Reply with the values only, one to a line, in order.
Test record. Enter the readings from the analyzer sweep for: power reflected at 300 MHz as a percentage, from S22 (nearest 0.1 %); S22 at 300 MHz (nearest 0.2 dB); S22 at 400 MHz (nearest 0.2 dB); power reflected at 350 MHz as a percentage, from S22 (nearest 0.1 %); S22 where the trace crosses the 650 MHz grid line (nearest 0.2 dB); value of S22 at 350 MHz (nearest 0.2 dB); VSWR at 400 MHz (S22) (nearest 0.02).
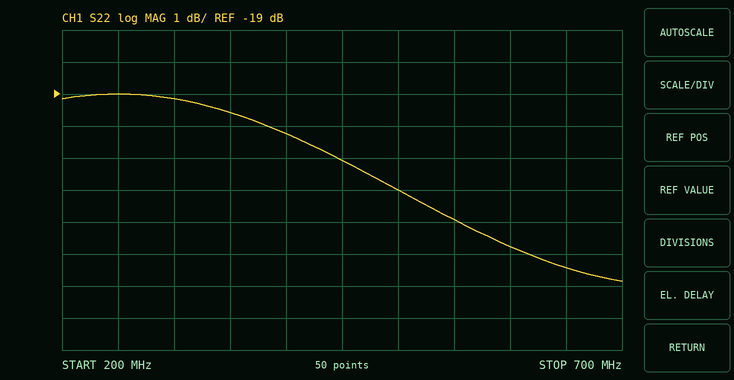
1.2 %
-19.2 dB
-20.2 dB
1.1 %
-24.4 dB
-19.6 dB
1.22
